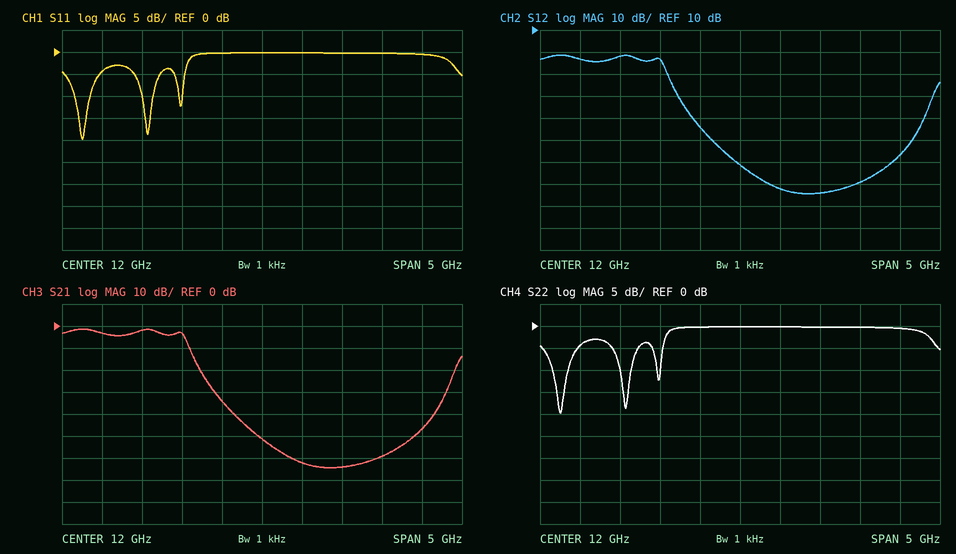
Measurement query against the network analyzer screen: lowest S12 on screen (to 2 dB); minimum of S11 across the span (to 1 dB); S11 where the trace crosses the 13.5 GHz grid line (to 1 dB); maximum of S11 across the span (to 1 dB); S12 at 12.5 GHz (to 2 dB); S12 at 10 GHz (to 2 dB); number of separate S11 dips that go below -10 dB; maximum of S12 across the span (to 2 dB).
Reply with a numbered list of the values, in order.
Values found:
1. -64 dB
2. -20 dB
3. 0 dB
4. 0 dB
5. -62 dB
6. -4 dB
7. 3
8. -2 dB
